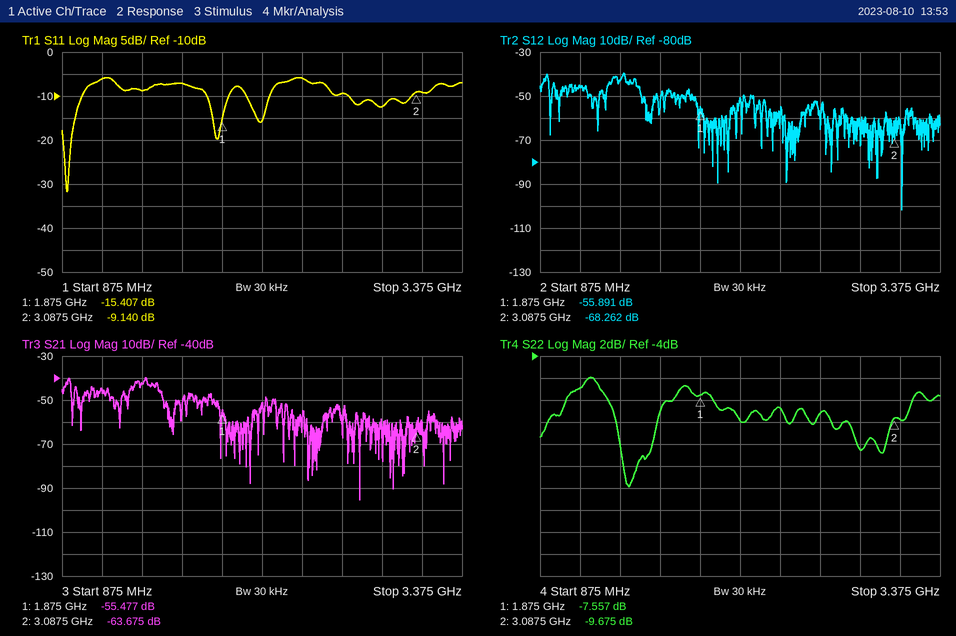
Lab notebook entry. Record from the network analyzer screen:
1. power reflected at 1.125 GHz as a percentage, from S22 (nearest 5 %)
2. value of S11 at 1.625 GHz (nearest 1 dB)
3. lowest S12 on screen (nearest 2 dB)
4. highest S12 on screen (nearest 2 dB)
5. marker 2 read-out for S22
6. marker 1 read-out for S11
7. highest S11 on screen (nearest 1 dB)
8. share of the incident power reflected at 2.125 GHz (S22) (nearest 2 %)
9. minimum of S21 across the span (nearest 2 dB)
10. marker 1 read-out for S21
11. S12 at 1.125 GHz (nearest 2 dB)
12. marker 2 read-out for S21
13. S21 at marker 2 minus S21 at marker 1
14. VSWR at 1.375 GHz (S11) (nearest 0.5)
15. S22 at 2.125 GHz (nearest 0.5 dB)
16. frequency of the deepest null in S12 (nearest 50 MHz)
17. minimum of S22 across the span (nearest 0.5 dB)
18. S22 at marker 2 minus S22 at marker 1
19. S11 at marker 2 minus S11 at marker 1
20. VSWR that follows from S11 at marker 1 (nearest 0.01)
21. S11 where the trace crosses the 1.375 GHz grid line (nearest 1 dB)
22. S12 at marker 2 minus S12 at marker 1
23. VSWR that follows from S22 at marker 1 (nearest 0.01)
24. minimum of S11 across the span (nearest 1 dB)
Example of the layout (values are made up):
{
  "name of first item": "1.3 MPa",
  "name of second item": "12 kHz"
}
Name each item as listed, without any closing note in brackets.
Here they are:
{
  "power reflected at 1.125 GHz as a percentage, from S22": "20 %",
  "value of S11 at 1.625 GHz": "-7 dB",
  "lowest S12 on screen": "-102 dB",
  "highest S12 on screen": "-40 dB",
  "marker 2 read-out for S22": "-9.675 dB",
  "marker 1 read-out for S11": "-15.407 dB",
  "highest S11 on screen": "-6 dB",
  "share of the incident power reflected at 2.125 GHz (S22)": "10 %",
  "minimum of S21 across the span": "-96 dB",
  "marker 1 read-out for S21": "-55.477 dB",
  "S12 at 1.125 GHz": "-46 dB",
  "marker 2 read-out for S21": "-63.675 dB",
  "S21 at marker 2 minus S21 at marker 1": "-8.198 dB",
  "VSWR at 1.375 GHz (S11)": "2.0",
  "S22 at 2.125 GHz": "-10.0 dB",
  "frequency of the deepest null in S12": "3.15 GHz",
  "minimum of S22 across the span": "-16.0 dB",
  "S22 at marker 2 minus S22 at marker 1": "-2.118 dB",
  "S11 at marker 2 minus S11 at marker 1": "6.267 dB",
  "VSWR that follows from S11 at marker 1": "1.41",
  "S11 where the trace crosses the 1.375 GHz grid line": "-9 dB",
  "S12 at marker 2 minus S12 at marker 1": "-12.371 dB",
  "VSWR that follows from S22 at marker 1": "2.44",
  "minimum of S11 across the span": "-32 dB"
}
